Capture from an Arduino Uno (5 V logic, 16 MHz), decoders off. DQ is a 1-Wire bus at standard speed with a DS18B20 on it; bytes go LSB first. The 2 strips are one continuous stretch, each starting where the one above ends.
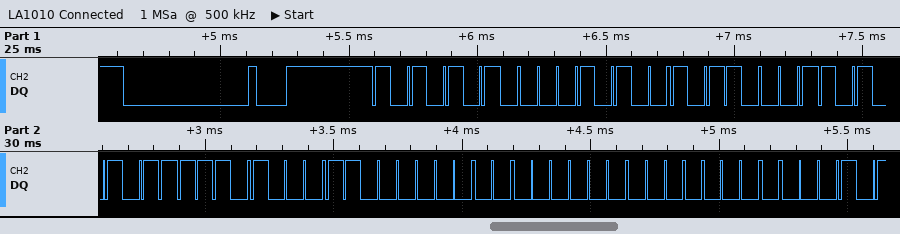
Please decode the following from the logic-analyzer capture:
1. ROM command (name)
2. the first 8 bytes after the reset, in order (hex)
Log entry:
Match ROM
55 28 8D D5 17 03 00 00
